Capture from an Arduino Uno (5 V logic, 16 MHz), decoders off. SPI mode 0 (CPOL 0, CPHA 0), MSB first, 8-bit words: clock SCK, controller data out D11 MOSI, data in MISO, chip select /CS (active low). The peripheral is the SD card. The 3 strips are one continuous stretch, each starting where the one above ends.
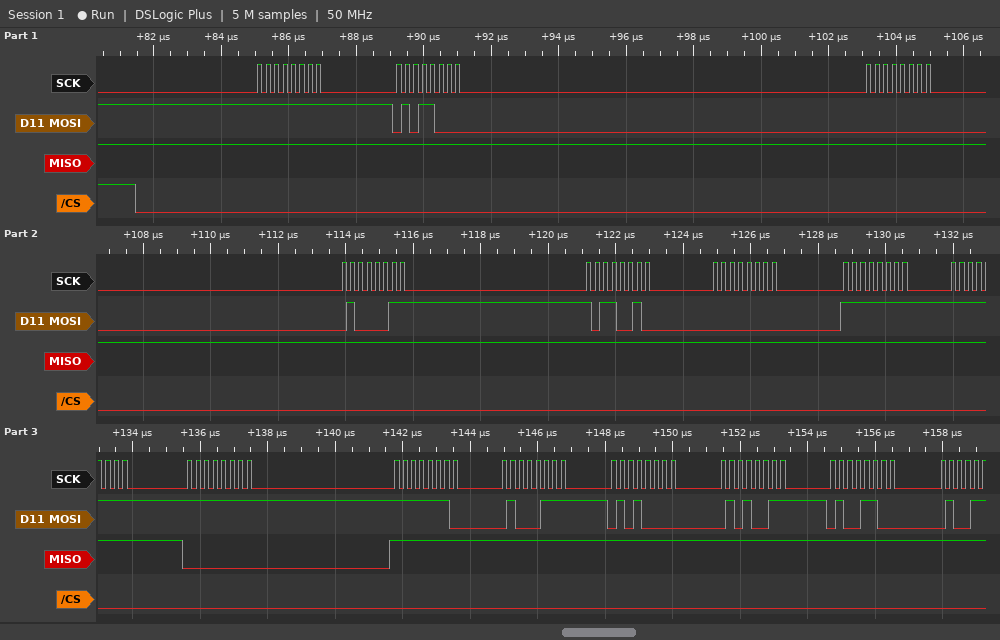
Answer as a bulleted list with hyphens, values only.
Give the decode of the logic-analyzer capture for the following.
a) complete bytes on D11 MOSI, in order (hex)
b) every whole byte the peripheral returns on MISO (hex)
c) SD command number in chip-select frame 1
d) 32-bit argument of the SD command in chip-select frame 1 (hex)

- FF 58 00 43 B2 00 FF FF FF FE 47 50 53 4C
- FF FF FF FF FF FF FF FF 00 FF FF FF FF FF
- CMD24
- 0x0043B200
